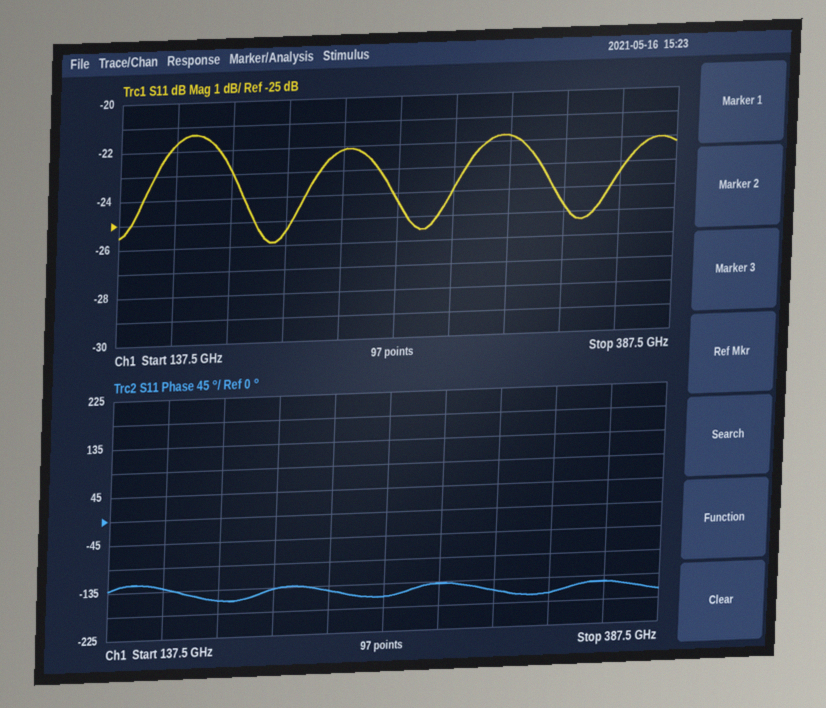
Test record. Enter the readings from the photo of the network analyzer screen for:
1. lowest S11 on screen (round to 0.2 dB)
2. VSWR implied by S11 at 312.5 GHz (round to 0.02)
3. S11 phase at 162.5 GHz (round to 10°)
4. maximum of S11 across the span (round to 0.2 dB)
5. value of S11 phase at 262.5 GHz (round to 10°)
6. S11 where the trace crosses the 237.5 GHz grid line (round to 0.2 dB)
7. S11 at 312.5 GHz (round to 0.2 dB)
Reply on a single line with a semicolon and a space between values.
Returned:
-25.8 dB; 1.18; -130°; -21.4 dB; -160°; -22.2 dB; -21.8 dB
